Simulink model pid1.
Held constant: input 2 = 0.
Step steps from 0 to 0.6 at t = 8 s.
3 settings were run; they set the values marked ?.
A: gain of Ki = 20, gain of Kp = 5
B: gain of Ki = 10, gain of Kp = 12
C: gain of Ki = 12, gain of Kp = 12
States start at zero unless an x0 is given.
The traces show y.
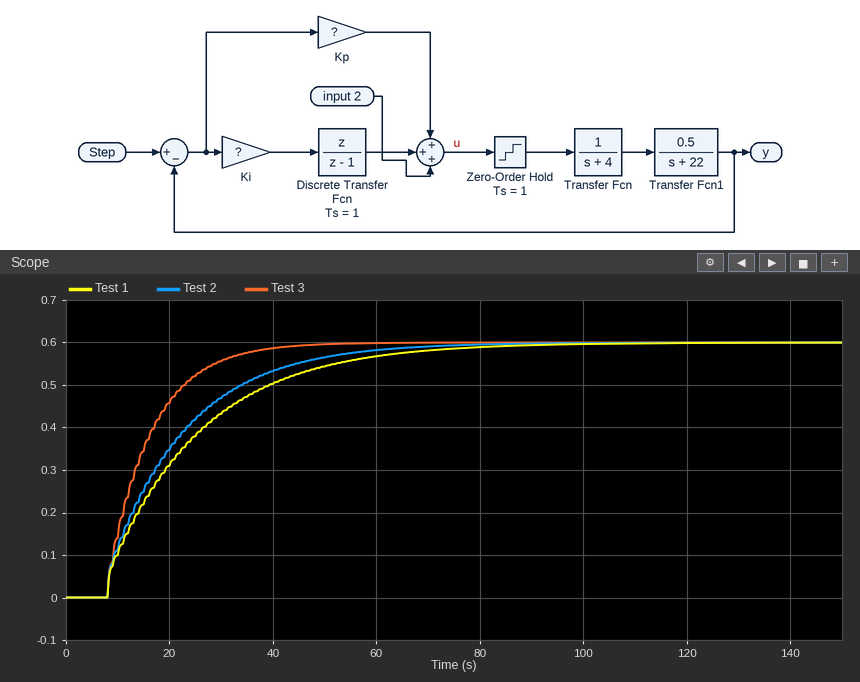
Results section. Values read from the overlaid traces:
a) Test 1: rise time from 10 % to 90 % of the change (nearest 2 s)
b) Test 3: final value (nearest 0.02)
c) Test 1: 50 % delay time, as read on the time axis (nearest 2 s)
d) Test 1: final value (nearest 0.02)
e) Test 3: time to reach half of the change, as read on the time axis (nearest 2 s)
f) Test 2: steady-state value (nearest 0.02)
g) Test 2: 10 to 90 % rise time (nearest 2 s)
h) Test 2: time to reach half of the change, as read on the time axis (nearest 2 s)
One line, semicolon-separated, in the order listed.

40 s; 0.60; 20 s; 0.60; 14 s; 0.60; 34 s; 18 s
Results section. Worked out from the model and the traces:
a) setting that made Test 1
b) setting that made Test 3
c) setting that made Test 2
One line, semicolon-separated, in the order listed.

B; A; C
